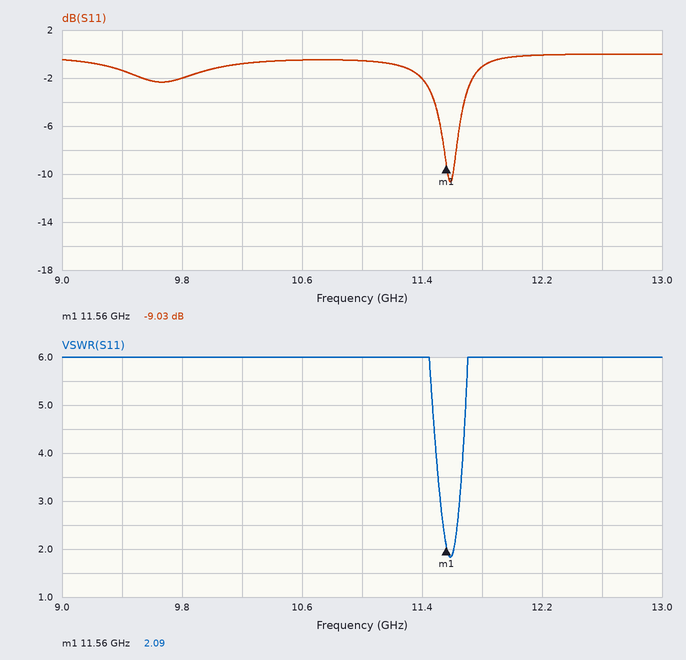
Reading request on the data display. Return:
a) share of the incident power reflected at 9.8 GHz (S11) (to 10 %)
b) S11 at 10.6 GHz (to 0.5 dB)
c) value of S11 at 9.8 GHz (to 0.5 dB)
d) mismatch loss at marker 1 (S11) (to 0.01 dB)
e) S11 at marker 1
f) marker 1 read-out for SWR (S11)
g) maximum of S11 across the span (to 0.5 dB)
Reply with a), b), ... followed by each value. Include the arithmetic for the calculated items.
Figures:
a) 10^(-2/10) ≈ 63.1 %, so 60 % to the nearest 10 %
b) -0.5 dB
c) -2.0 dB
d) −10 log10(1 − 10^(-9.03/10)) ≈ 0.58 dB
e) -9.03 dB
f) 2.09
g) 0.0 dB
